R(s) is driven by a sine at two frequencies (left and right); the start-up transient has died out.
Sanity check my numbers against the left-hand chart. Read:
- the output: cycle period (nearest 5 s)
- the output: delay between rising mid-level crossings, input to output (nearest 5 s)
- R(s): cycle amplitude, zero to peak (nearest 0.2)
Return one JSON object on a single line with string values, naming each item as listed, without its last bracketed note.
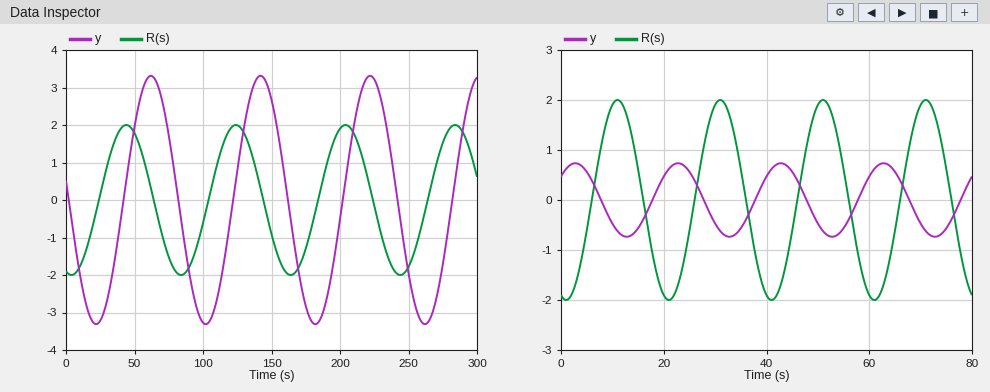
{"the output: cycle period": "80 s", "the output: delay between rising mid-level crossings, input to output": "20 s", "R(s): cycle amplitude, zero to peak": "2.0"}
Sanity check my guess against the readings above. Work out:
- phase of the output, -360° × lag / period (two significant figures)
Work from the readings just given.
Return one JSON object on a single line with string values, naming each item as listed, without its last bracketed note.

{"phase of the output, -360° × lag / period": "-90°"}
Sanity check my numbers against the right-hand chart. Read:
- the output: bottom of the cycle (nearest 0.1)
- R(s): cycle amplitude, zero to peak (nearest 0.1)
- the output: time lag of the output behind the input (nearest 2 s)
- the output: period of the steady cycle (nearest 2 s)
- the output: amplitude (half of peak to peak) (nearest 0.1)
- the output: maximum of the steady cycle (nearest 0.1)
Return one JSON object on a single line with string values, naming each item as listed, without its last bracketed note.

{"the output: bottom of the cycle": "-0.7", "R(s): cycle amplitude, zero to peak": "2.0", "the output: time lag of the output behind the input": "12 s", "the output: period of the steady cycle": "20 s", "the output: amplitude (half of peak to peak)": "0.7", "the output: maximum of the steady cycle": "0.7"}
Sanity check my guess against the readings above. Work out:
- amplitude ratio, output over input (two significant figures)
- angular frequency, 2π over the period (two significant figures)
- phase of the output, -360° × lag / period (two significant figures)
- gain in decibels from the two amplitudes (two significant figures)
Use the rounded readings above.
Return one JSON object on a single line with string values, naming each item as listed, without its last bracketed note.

{"amplitude ratio, output over input": "0.35", "angular frequency, 2π over the period": "0.31 rad/s", "phase of the output, -360° × lag / period": "-220°", "gain in decibels from the two amplitudes": "-9.1 dB"}
